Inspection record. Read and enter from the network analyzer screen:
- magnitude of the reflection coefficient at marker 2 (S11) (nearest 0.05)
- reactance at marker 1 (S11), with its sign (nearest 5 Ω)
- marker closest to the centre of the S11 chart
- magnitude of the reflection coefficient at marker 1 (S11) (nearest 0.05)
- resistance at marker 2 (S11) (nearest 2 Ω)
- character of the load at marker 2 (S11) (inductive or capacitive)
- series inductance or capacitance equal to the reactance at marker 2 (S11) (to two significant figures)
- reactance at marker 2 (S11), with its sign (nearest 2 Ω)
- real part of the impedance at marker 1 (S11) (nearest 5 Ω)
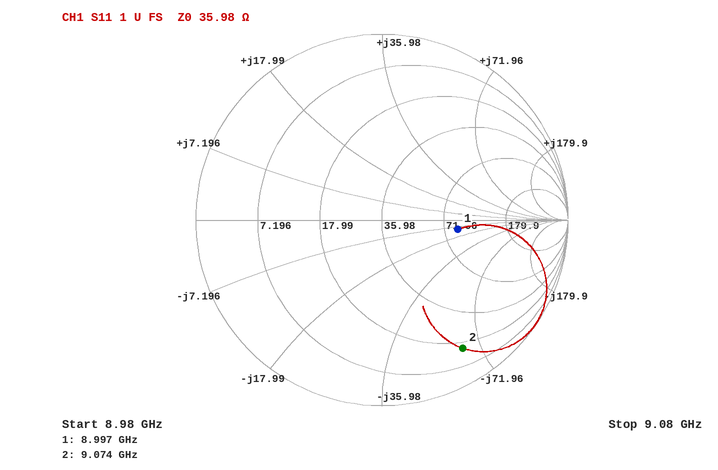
0.80
-10 Ω
marker 1
0.40
16 Ω
capacitive
280 fF
-62 Ω
85 Ω
